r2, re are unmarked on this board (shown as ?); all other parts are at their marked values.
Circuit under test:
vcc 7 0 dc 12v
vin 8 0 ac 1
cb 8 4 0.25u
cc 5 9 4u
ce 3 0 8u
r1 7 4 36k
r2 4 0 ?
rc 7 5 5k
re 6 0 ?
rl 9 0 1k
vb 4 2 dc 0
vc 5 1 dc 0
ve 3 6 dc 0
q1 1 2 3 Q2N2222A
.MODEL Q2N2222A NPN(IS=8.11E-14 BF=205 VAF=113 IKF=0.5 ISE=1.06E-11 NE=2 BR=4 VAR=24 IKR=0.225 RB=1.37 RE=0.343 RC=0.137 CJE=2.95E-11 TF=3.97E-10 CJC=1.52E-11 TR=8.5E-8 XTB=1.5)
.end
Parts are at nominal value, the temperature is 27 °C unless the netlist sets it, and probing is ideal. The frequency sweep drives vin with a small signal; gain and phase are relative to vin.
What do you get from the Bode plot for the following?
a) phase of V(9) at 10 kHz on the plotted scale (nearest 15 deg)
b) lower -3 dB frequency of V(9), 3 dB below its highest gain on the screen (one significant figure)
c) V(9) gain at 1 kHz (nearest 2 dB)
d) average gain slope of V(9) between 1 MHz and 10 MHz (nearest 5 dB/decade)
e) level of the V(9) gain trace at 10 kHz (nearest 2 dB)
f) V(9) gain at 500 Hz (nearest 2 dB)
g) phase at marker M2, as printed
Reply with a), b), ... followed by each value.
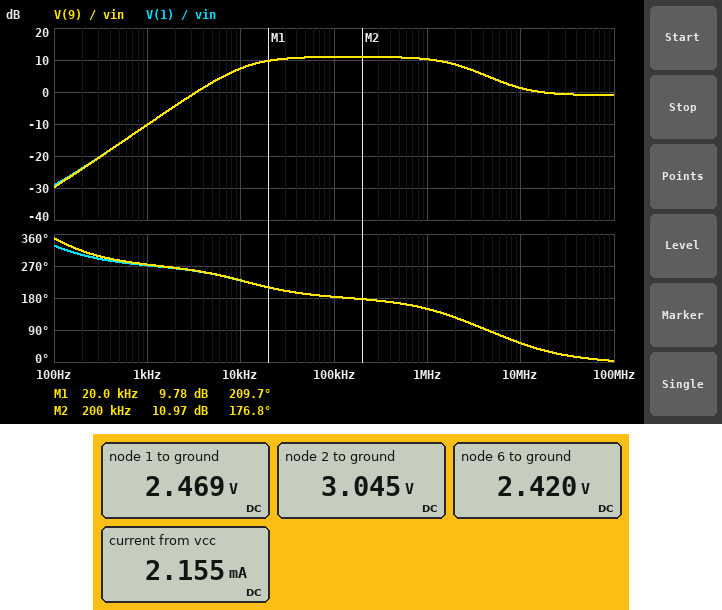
a) 225 deg
b) 10 kHz
c) -10 dB
d) -10 dB/decade
e) 8 dB
f) -16 dB
g) 176.8 deg
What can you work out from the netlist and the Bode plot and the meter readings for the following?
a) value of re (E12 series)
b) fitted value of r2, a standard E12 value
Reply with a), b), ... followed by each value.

a) 1.2 kΩ
b) 22 kΩ
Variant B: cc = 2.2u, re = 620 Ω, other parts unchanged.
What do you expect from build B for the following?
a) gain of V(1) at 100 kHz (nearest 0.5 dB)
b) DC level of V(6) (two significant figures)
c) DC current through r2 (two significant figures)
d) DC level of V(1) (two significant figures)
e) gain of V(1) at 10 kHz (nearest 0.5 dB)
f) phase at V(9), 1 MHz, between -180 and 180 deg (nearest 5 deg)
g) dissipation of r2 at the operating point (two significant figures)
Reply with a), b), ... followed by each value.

a) 7.0 dB
b) 1.4 V
c) 93 µA
d) 1.5 V
e) 2.5 dB
f) 145 deg
g) 190 µW
